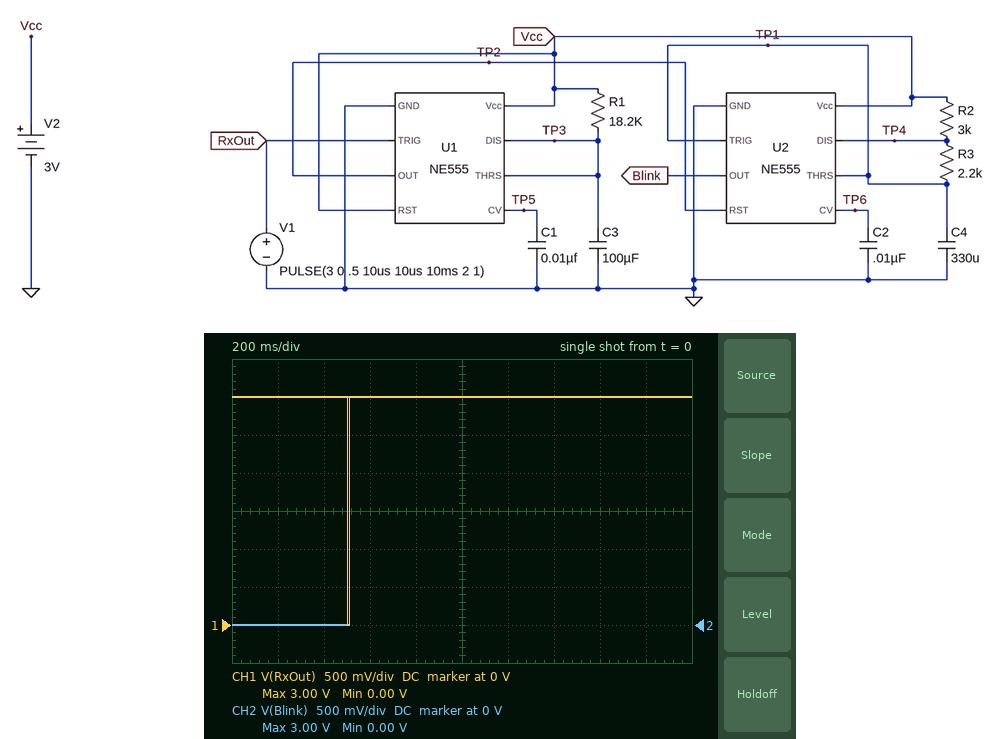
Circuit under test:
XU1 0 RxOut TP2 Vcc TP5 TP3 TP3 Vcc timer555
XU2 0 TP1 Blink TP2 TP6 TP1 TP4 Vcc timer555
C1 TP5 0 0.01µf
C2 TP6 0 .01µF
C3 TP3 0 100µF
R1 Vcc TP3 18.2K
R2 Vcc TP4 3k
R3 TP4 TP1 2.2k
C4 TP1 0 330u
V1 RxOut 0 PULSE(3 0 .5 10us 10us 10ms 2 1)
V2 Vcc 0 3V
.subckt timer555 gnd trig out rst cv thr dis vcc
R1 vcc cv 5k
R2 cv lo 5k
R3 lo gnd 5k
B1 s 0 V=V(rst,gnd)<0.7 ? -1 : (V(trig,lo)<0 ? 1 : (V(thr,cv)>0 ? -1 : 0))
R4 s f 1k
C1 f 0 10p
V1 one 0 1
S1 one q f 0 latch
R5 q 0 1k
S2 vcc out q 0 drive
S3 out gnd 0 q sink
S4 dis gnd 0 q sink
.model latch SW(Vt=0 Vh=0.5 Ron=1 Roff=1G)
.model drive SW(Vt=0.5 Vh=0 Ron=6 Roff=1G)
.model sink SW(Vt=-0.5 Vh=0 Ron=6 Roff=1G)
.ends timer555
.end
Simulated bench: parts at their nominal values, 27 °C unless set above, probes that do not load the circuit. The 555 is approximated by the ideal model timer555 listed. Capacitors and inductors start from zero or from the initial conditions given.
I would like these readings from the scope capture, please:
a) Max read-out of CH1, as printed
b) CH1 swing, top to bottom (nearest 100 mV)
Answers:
3.00 V
3.0 V
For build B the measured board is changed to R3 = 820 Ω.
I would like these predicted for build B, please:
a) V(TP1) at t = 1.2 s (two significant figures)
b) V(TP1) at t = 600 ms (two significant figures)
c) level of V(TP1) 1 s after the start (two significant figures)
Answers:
1.3 V
230 mV
990 mV
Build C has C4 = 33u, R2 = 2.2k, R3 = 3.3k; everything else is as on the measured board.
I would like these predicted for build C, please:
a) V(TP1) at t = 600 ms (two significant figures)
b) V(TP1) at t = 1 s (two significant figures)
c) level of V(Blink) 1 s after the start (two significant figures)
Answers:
1.3 V
1.2 V
3.0 V
